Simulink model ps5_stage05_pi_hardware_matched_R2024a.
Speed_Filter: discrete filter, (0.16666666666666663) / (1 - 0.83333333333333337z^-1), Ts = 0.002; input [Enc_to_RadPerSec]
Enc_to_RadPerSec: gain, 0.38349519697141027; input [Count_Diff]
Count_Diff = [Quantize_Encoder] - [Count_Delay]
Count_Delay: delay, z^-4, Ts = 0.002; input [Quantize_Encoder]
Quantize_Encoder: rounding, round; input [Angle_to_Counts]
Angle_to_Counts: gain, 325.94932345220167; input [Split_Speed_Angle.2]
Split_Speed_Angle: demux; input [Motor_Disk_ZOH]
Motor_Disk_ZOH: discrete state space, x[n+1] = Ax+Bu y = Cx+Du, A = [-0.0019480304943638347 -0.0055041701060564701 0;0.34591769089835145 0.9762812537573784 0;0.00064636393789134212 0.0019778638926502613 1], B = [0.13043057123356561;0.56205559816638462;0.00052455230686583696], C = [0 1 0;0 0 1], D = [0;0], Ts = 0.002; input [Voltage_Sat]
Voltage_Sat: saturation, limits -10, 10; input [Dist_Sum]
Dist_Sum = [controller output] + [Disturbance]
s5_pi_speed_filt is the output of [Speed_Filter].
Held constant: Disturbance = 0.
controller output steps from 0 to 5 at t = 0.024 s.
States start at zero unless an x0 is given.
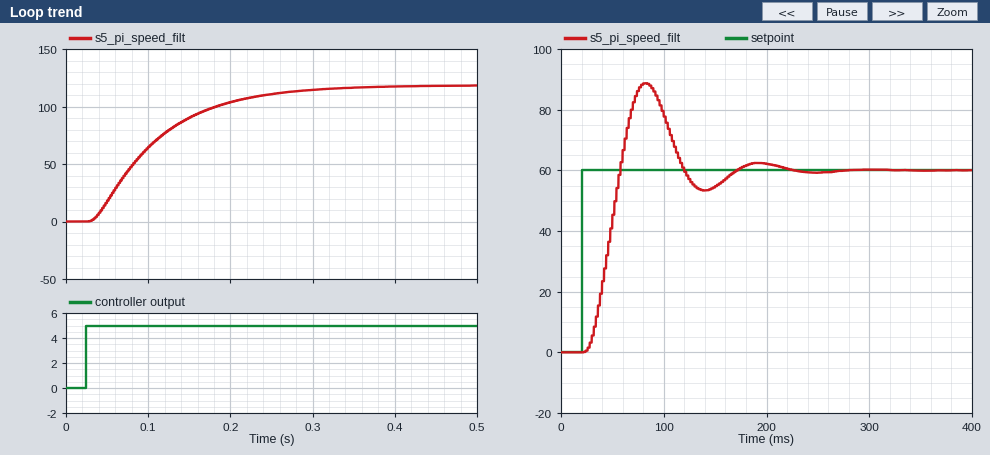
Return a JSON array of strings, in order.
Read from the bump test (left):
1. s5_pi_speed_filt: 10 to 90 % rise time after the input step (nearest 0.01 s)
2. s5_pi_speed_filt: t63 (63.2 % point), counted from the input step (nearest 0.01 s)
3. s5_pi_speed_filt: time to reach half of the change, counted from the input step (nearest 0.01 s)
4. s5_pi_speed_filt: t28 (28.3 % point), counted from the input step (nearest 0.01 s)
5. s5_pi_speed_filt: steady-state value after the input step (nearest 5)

["0.17 s", "0.09 s", "0.07 s", "0.04 s", "120"]
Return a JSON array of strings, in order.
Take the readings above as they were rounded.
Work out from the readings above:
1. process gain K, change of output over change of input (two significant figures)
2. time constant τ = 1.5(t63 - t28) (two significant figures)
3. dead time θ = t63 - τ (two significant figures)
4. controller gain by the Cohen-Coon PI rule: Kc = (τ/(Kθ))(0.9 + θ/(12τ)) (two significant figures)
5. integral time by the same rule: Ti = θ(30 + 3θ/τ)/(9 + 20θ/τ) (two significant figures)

["24", "0.075 s", "0.015 s", "0.19", "0.035 s"]
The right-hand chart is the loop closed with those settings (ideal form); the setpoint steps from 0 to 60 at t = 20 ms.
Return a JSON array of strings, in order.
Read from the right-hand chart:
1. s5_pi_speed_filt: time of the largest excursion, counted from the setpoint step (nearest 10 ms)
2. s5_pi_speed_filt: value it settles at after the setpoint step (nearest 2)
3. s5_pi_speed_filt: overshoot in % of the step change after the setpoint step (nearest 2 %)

["60 ms", "60", "48 %"]
